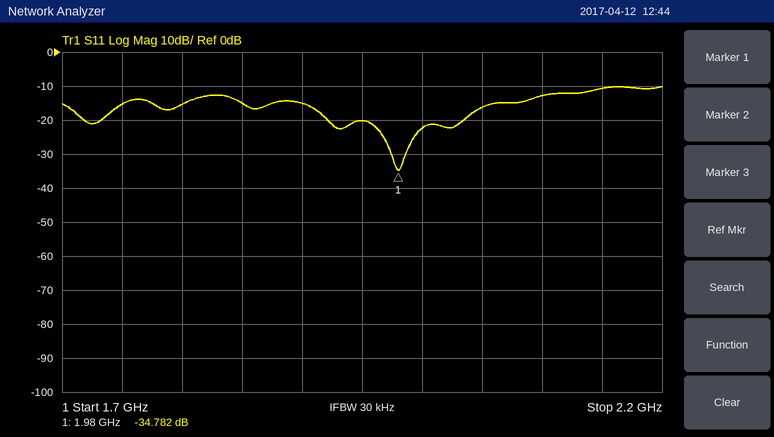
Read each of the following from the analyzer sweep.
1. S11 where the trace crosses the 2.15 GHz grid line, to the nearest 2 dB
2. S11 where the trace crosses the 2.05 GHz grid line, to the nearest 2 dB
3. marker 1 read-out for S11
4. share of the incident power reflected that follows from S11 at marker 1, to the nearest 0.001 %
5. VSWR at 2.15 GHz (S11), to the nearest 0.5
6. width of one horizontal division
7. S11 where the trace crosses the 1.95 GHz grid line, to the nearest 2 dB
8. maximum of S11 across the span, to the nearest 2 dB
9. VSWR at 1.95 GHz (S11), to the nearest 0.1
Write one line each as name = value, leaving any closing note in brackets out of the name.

S11 where the trace crosses the 2.15 GHz grid line, to the nearest 2 dB = -10 dB
S11 where the trace crosses the 2.05 GHz grid line, to the nearest 2 dB = -16 dB
marker 1 read-out for S11 = -34.782 dB
share of the incident power reflected that follows from S11 at marker 1, to the nearest 0.001 % = 0.033 %
VSWR at 2.15 GHz (S11), to the nearest 0.5 = 2.0
width of one horizontal division = 50 MHz
S11 where the trace crosses the 1.95 GHz grid line, to the nearest 2 dB = -20 dB
maximum of S11 across the span, to the nearest 2 dB = -10 dB
VSWR at 1.95 GHz (S11), to the nearest 0.1 = 1.2
